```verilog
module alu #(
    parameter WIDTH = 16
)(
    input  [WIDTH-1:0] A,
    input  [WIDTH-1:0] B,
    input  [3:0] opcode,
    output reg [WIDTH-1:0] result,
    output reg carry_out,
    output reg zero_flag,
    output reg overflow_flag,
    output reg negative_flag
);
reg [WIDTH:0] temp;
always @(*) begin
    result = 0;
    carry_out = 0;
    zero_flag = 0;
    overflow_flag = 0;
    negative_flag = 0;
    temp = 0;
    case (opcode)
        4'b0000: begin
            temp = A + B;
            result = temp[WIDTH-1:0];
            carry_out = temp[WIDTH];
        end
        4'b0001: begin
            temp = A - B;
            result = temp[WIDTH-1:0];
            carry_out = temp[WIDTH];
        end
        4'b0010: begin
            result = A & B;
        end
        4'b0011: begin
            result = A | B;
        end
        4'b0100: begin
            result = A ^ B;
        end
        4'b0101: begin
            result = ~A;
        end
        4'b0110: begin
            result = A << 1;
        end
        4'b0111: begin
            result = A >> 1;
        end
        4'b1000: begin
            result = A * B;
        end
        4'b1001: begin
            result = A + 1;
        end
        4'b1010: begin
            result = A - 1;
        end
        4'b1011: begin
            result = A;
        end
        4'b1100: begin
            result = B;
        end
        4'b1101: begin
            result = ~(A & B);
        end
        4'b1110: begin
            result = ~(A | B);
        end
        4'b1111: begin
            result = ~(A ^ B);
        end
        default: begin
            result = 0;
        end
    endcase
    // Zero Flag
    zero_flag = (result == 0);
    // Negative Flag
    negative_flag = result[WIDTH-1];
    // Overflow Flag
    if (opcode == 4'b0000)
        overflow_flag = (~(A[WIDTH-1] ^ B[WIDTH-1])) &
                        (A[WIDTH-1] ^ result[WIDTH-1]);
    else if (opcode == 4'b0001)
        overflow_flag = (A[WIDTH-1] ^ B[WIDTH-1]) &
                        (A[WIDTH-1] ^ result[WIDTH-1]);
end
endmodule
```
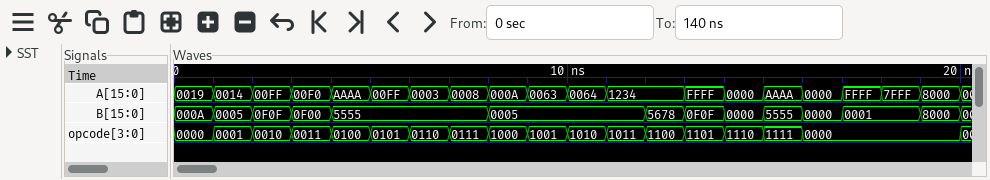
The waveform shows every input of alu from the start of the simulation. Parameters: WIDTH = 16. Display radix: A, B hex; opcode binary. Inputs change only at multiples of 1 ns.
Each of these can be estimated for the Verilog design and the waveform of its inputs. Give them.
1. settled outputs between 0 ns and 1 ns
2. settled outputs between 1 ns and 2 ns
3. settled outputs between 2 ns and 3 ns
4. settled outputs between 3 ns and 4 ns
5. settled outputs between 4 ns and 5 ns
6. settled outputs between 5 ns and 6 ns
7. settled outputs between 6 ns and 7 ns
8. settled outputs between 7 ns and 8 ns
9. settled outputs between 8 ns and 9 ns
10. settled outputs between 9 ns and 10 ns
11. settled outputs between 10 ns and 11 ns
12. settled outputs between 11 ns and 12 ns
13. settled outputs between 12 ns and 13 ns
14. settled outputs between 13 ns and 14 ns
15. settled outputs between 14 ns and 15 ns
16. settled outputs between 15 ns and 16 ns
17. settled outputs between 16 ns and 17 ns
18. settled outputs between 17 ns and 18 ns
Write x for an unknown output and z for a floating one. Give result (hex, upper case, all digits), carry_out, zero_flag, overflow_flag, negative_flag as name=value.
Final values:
result=0023, carry_out=0, zero_flag=0, overflow_flag=0, negative_flag=0
result=000F, carry_out=0, zero_flag=0, overflow_flag=0, negative_flag=0
result=000F, carry_out=0, zero_flag=0, overflow_flag=0, negative_flag=0
result=0FF0, carry_out=0, zero_flag=0, overflow_flag=0, negative_flag=0
result=FFFF, carry_out=0, zero_flag=0, overflow_flag=0, negative_flag=1
result=FF00, carry_out=0, zero_flag=0, overflow_flag=0, negative_flag=1
result=0006, carry_out=0, zero_flag=0, overflow_flag=0, negative_flag=0
result=0004, carry_out=0, zero_flag=0, overflow_flag=0, negative_flag=0
result=0032, carry_out=0, zero_flag=0, overflow_flag=0, negative_flag=0
result=0064, carry_out=0, zero_flag=0, overflow_flag=0, negative_flag=0
result=0063, carry_out=0, zero_flag=0, overflow_flag=0, negative_flag=0
result=1234, carry_out=0, zero_flag=0, overflow_flag=0, negative_flag=0
result=5678, carry_out=0, zero_flag=0, overflow_flag=0, negative_flag=0
result=F0F0, carry_out=0, zero_flag=0, overflow_flag=0, negative_flag=1
result=FFFF, carry_out=0, zero_flag=0, overflow_flag=0, negative_flag=1
result=0000, carry_out=0, zero_flag=1, overflow_flag=0, negative_flag=0
result=0000, carry_out=0, zero_flag=1, overflow_flag=0, negative_flag=0
result=0000, carry_out=1, zero_flag=1, overflow_flag=0, negative_flag=0
